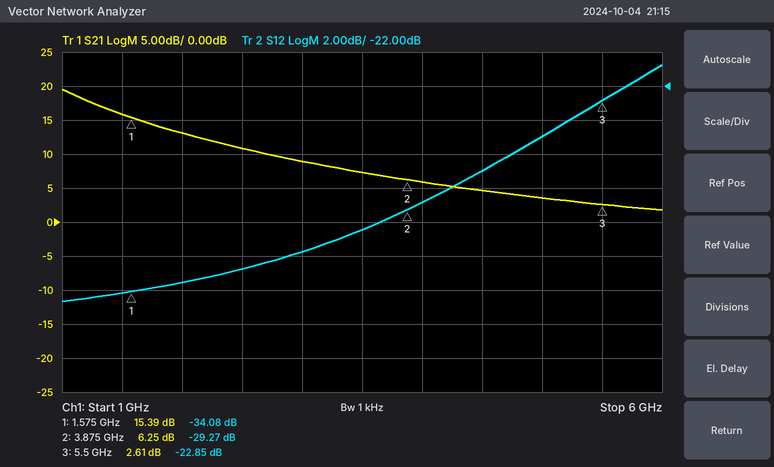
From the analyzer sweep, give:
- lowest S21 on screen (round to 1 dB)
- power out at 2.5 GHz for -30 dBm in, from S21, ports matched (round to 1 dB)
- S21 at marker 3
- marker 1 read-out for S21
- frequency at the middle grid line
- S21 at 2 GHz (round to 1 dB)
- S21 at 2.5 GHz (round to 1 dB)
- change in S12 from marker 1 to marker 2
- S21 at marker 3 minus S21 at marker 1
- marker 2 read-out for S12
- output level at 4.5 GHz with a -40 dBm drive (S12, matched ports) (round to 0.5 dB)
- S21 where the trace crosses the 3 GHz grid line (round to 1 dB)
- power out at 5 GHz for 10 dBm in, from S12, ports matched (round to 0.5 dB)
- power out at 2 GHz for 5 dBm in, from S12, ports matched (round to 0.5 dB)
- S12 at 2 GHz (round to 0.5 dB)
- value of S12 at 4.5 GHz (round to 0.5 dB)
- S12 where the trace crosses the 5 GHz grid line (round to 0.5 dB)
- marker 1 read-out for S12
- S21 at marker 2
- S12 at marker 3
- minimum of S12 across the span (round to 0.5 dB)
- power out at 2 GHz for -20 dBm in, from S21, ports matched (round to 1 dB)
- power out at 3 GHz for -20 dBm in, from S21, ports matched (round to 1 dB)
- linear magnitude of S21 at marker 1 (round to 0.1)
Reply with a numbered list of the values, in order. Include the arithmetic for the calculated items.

1. 2 dB
2. -30 dBm + (11 dB) = -19 dBm
3. 2.61 dB
4. 15.39 dB
5. 3.5 GHz
6. 13 dB
7. 11 dB
8. -29.27 − (-34.08) = 4.81 dB
9. 2.61 − (15.39) = -12.78 dB
10. -29.27 dB
11. -40 dBm + (-27.0 dB) = -67.0 dBm
12. 9 dB
13. 10 dBm + (-25.0 dB) = -15.0 dBm
14. 5 dBm + (-33.5 dB) = -28.5 dBm
15. -33.5 dB
16. -27.0 dB
17. -25.0 dB
18. -34.08 dB
19. 6.25 dB
20. -22.85 dB
21. -34.5 dB
22. -20 dBm + (13 dB) = -7 dBm
23. -20 dBm + (9 dB) = -11 dBm
24. 10^(15.39/20) ≈ 5.9
